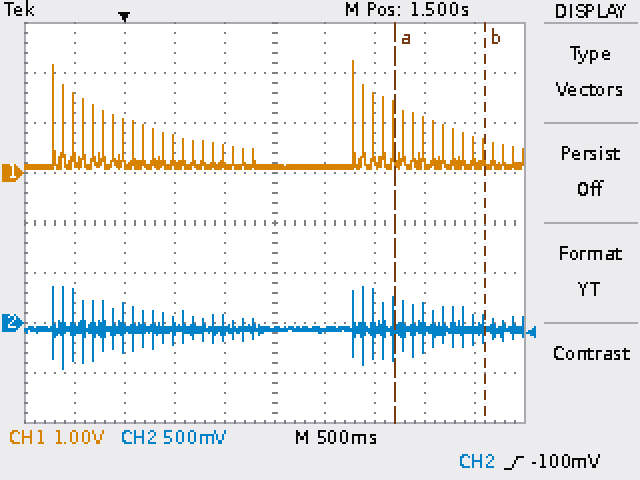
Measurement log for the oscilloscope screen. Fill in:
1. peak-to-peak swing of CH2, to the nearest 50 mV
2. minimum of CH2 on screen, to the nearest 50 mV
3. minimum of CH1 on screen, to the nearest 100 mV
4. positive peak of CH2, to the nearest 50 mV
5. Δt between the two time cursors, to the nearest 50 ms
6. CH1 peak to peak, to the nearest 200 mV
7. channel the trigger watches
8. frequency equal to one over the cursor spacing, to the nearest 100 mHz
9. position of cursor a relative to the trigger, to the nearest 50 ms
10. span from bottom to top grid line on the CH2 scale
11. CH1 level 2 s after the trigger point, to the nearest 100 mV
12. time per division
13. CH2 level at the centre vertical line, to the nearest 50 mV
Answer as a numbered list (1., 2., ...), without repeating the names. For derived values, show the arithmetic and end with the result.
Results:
1. 350 mV − (-450 mV) = 800 mV
2. -450 mV
3. 100 mV
4. 350 mV
5. 900 ms
6. 2.2 V
7. CH2
8. 1 / 900 ms ≈ 1.1 Hz
9. +2.70 s
10. 4 V
11. 100 mV
12. 500 ms
13. -50 mV
